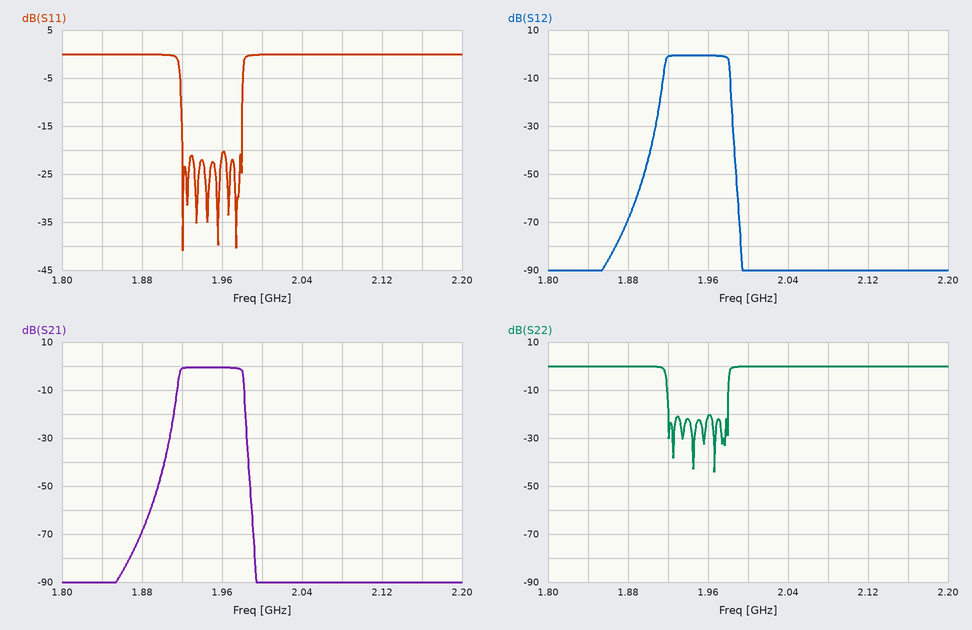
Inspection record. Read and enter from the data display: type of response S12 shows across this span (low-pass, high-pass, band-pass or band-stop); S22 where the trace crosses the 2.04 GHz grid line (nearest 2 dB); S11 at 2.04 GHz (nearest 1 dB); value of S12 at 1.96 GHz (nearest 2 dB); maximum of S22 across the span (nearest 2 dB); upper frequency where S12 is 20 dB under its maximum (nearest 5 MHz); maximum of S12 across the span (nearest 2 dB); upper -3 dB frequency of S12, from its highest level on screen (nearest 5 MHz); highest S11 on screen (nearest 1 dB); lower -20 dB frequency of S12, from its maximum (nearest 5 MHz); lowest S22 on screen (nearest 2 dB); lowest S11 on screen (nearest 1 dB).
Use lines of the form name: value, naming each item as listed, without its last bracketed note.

type of response S12 shows across this span: band-pass
S22 where the trace crosses the 2.04 GHz grid line: 0 dB
S11 at 2.04 GHz: 0 dB
value of S12 at 1.96 GHz: 0 dB
maximum of S22 across the span: 0 dB
upper frequency where S12 is 20 dB under its maximum: 1.985 GHz
maximum of S12 across the span: 0 dB
upper -3 dB frequency of S12, from its highest level on screen: 1.980 GHz
highest S11 on screen: 0 dB
lower -20 dB frequency of S12, from its maximum: 1.910 GHz
lowest S22 on screen: -44 dB
lowest S11 on screen: -41 dB
